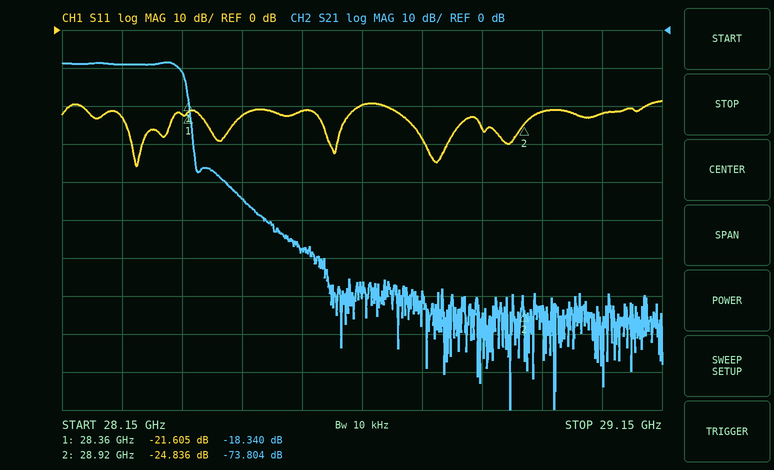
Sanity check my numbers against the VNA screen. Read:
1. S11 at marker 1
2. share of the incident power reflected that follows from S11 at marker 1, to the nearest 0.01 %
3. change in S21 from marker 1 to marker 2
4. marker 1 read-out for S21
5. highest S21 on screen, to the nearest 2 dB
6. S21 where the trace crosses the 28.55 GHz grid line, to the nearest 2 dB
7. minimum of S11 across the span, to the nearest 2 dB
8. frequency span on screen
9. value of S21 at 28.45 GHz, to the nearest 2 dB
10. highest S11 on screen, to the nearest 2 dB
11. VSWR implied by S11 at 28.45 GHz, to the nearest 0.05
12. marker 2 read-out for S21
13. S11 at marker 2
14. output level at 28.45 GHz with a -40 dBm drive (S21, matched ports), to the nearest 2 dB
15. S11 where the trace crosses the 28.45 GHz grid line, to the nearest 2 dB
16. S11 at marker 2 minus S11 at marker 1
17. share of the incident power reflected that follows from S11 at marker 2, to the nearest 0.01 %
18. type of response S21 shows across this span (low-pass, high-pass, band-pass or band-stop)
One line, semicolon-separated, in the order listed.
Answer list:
-21.605 dB; 0.69 %; -55.464 dB; -18.340 dB; -8 dB; -58 dB; -36 dB; 1 GHz; -44 dB; -18 dB; 1.15; -73.804 dB; -24.836 dB; -84 dBm; -22 dB; -3.231 dB; 0.33 %; low-pass
